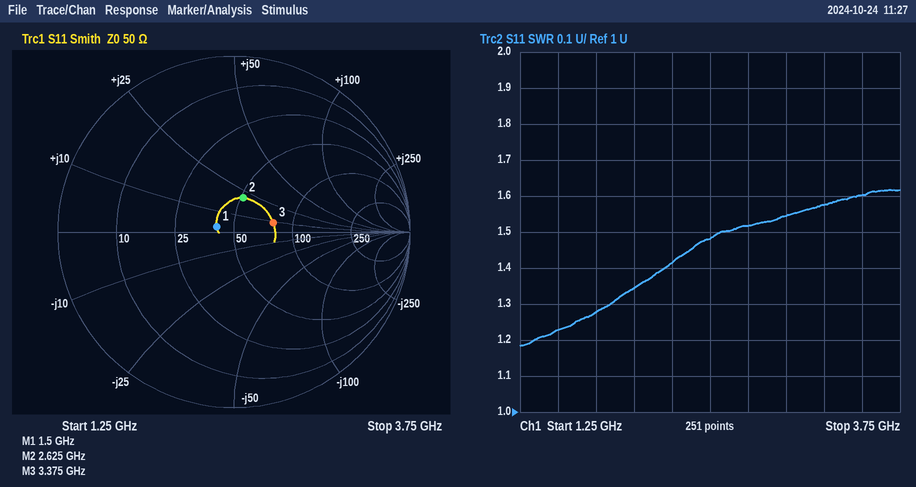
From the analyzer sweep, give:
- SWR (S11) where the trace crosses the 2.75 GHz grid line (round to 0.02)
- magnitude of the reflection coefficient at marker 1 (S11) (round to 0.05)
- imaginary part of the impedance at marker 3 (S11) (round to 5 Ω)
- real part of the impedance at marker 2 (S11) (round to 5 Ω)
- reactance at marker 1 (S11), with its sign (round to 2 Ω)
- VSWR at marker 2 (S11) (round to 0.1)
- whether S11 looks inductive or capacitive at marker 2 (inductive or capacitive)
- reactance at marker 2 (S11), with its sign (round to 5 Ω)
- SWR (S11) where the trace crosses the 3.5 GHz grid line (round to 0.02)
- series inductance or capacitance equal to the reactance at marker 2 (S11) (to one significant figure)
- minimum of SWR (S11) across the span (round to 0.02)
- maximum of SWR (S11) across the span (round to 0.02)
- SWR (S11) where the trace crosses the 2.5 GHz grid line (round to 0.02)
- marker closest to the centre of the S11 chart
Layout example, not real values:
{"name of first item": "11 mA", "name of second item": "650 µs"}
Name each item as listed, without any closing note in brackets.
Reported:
{"SWR (S11) where the trace crosses the 2.75 GHz grid line": "1.52", "magnitude of the reflection coefficient at marker 1 (S11)": "0.10", "imaginary part of the impedance at marker 3 (S11)": "+10 Ω", "real part of the impedance at marker 2 (S11)": "50 Ω", "reactance at marker 1 (S11), with its sign": "+2 Ω", "VSWR at marker 2 (S11)": "1.5", "whether S11 looks inductive or capacitive at marker 2": "inductive", "reactance at marker 2 (S11), with its sign": "+20 Ω", "SWR (S11) where the trace crosses the 3.5 GHz grid line": "1.60", "series inductance or capacitance equal to the reactance at marker 2 (S11)": "1 nH", "minimum of SWR (S11) across the span": "1.18", "maximum of SWR (S11) across the span": "1.62", "SWR (S11) where the trace crosses the 2.5 GHz grid line": "1.48", "marker closest to the centre of the S11 chart": "marker 1"}
